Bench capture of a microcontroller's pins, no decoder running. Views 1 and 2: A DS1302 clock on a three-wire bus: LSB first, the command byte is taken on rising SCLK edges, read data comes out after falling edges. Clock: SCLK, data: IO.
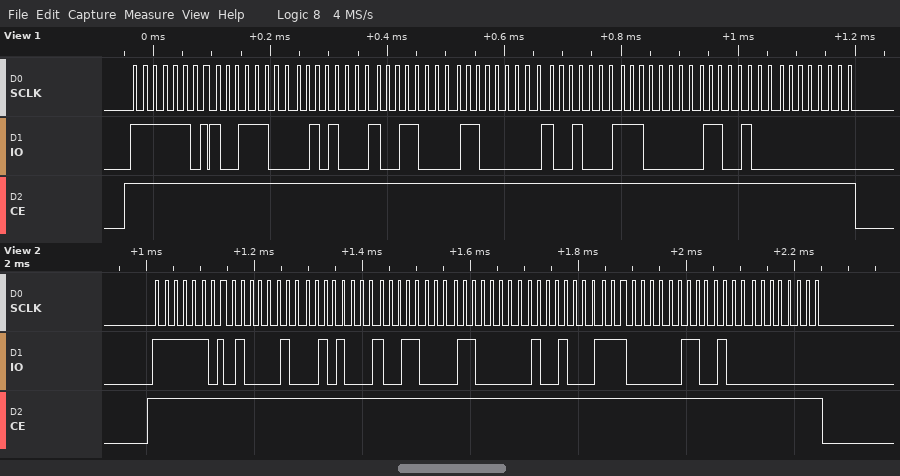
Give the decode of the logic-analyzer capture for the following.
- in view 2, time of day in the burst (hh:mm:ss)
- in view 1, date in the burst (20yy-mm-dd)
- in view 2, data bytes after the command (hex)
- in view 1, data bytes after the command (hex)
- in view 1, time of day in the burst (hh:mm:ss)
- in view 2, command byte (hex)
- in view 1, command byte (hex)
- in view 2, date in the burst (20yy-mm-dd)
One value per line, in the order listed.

19:14:42
2026-12-06
42 14 19 06 12 07 26 00
39 14 19 06 12 07 26 00
19:14:39
0xBF
0xBF
2026-12-06
